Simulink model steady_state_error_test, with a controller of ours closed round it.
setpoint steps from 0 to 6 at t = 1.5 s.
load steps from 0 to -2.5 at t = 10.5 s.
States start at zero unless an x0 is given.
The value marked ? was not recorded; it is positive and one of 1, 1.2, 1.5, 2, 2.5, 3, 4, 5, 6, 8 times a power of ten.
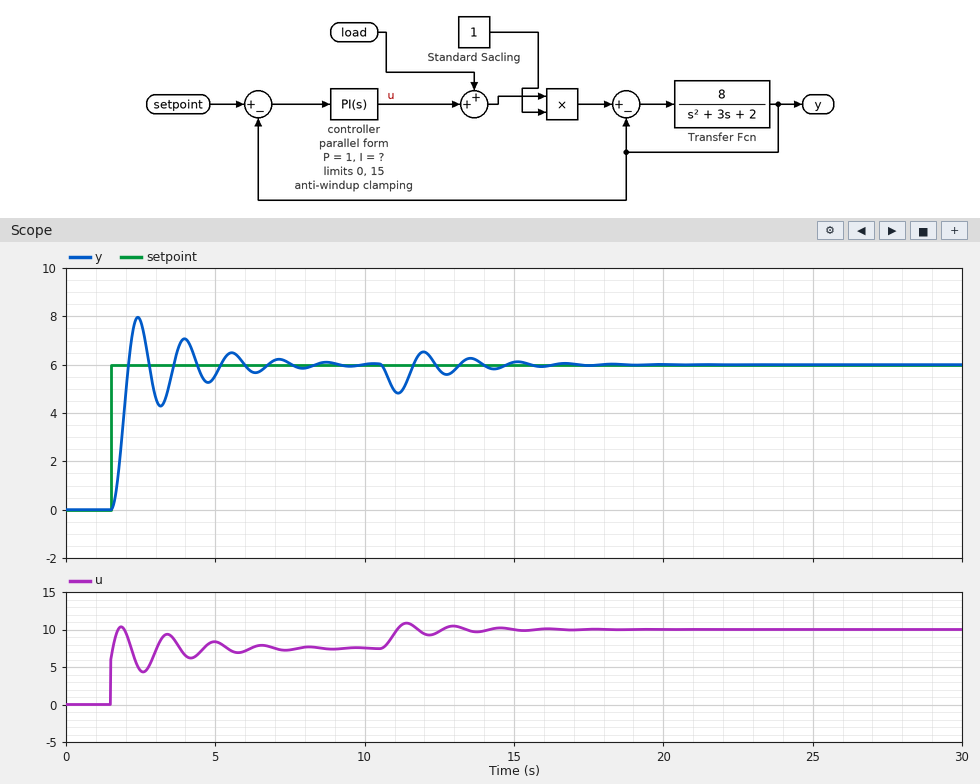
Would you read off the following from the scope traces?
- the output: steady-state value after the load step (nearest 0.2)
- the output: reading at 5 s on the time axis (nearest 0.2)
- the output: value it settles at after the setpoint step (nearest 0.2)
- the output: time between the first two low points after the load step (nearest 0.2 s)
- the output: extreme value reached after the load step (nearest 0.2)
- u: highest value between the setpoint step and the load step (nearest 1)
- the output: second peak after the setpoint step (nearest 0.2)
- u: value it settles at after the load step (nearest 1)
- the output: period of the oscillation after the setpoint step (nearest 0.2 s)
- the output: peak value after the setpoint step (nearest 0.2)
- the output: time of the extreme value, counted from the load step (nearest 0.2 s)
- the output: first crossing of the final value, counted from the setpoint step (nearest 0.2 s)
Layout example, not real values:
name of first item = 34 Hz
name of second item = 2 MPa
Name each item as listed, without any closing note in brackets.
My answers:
the output: steady-state value after the load step = 6.0
the output: reading at 5 s on the time axis = 5.6
the output: value it settles at after the setpoint step = 6.0
the output: time between the first two low points after the load step = 1.6 s
the output: extreme value reached after the load step = 4.8
u: highest value between the setpoint step and the load step = 10
the output: second peak after the setpoint step = 7.0
u: value it settles at after the load step = 10
the output: period of the oscillation after the setpoint step = 1.6 s
the output: peak value after the setpoint step = 8.0
the output: time of the extreme value, counted from the load step = 0.6 s
the output: first crossing of the final value, counted from the setpoint step = 0.6 s
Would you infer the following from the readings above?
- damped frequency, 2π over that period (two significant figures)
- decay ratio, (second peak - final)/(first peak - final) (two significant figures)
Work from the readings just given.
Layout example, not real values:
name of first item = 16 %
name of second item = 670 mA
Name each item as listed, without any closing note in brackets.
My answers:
damped frequency, 2π over that period = 3.9 rad/s
decay ratio, (second peak - final)/(first peak - final) = 0.50
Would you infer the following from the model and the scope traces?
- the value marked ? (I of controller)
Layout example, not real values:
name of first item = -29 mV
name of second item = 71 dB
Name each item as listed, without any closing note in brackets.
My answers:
the value marked ? = 4
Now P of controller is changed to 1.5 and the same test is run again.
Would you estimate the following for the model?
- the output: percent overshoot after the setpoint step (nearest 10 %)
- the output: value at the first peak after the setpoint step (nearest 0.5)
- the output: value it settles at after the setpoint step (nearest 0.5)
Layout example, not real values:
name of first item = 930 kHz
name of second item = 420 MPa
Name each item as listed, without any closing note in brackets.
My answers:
the output: percent overshoot after the setpoint step = 30 %
the output: value at the first peak after the setpoint step = 7.5
the output: value it settles at after the setpoint step = 6.0
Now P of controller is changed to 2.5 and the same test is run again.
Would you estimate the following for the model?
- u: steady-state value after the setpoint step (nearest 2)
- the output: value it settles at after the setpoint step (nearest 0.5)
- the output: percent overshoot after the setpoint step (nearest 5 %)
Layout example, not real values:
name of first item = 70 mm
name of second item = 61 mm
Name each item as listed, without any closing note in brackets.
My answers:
u: steady-state value after the setpoint step = 8
the output: value it settles at after the setpoint step = 6.0
the output: percent overshoot after the setpoint step = 20 %
